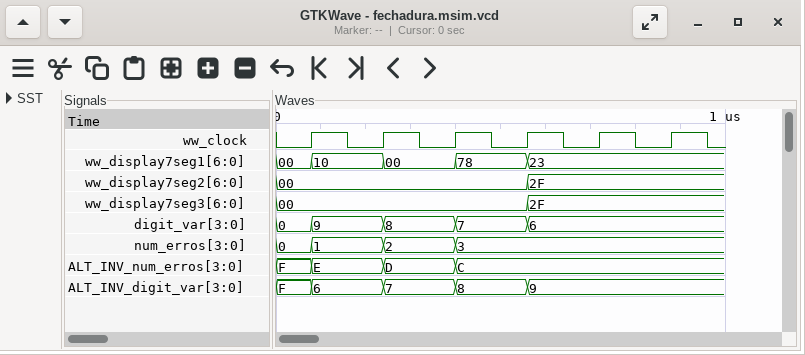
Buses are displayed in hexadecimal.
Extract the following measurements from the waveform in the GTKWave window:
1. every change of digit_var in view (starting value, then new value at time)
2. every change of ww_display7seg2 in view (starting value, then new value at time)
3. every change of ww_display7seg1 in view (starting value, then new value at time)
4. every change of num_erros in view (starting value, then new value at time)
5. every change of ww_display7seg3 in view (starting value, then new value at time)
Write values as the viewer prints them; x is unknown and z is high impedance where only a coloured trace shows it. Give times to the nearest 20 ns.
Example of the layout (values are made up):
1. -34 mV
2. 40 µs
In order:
1. 0, 9 at 80 ns, 8 at 240 ns, 7 at 400 ns, 6 at 560 ns
2. 00, 2F at 560 ns
3. 00, 10 at 80 ns, 00 at 240 ns, 78 at 400 ns, 23 at 560 ns
4. 0, 1 at 80 ns, 2 at 240 ns, 3 at 400 ns
5. 00, 2F at 560 ns
